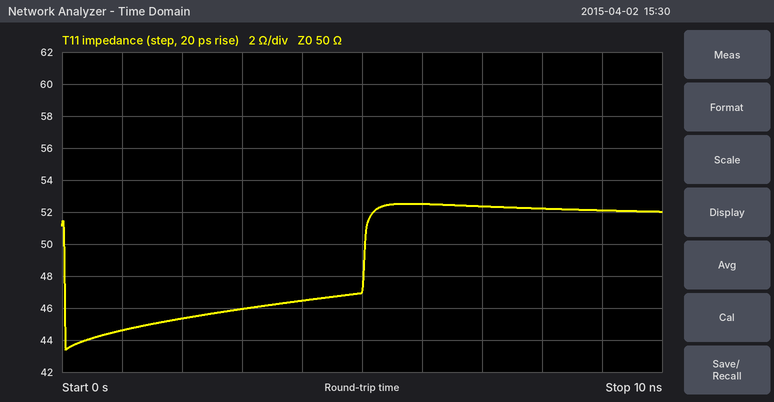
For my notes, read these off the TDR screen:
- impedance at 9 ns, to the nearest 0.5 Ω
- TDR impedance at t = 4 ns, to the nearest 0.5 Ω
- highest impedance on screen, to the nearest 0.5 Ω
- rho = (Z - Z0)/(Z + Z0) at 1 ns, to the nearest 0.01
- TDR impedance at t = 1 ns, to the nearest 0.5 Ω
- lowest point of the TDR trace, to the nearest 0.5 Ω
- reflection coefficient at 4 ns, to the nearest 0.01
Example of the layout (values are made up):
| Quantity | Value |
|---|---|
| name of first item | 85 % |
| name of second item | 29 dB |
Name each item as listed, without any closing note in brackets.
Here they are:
| Quantity | Value |
|---|---|
| impedance at 9 ns, to the nearest 0.5 Ω | 52.0 Ω |
| TDR impedance at t = 4 ns, to the nearest 0.5 Ω | 46.5 Ω |
| highest impedance on screen, to the nearest 0.5 Ω | 52.5 Ω |
| rho = (Z - Z0)/(Z + Z0) at 1 ns, to the nearest 0.01 | -0.06 |
| TDR impedance at t = 1 ns, to the nearest 0.5 Ω | 44.5 Ω |
| lowest point of the TDR trace, to the nearest 0.5 Ω | 43.5 Ω |
| reflection coefficient at 4 ns, to the nearest 0.01 | -0.04 |
